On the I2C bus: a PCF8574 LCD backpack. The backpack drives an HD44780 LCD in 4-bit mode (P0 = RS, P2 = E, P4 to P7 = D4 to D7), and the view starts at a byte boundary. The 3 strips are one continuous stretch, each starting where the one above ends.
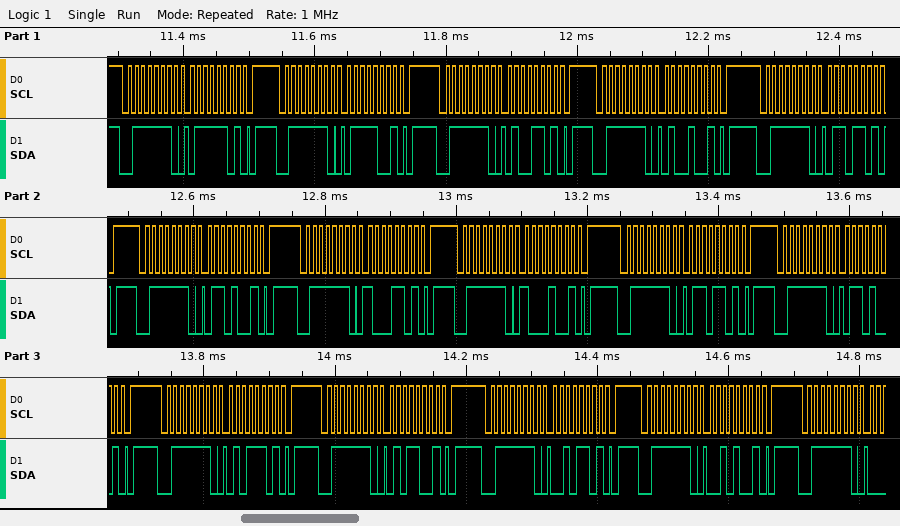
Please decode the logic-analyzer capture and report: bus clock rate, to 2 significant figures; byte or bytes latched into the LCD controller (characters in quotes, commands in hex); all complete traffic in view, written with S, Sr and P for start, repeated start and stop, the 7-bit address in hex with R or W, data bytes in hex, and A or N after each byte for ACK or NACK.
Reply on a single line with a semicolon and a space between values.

100 kHz; 't' 'h' 'e'; S 3FW A 7D A P S 3FW A 79 A P S 3FW A 4D A P S 3FW A 49 A P S 3FW A 6D A P S 3FW A 69 A P S 3FW A 8D A P S 3FW A 89 A P S 3FW A 6D A P S 3FW A 69 A P S 3FW A 5D A P S 3FW A 59 A P S 3FW A 2D A P S 3FW A 29 A P S 3FW A
